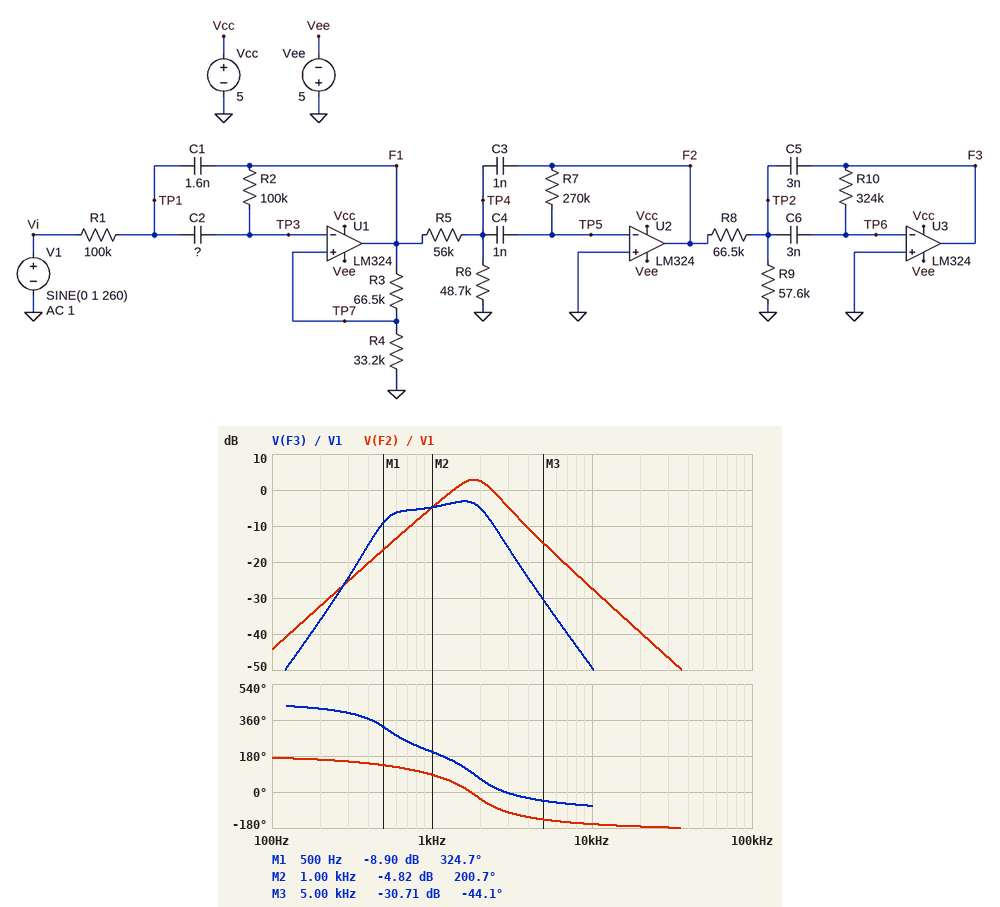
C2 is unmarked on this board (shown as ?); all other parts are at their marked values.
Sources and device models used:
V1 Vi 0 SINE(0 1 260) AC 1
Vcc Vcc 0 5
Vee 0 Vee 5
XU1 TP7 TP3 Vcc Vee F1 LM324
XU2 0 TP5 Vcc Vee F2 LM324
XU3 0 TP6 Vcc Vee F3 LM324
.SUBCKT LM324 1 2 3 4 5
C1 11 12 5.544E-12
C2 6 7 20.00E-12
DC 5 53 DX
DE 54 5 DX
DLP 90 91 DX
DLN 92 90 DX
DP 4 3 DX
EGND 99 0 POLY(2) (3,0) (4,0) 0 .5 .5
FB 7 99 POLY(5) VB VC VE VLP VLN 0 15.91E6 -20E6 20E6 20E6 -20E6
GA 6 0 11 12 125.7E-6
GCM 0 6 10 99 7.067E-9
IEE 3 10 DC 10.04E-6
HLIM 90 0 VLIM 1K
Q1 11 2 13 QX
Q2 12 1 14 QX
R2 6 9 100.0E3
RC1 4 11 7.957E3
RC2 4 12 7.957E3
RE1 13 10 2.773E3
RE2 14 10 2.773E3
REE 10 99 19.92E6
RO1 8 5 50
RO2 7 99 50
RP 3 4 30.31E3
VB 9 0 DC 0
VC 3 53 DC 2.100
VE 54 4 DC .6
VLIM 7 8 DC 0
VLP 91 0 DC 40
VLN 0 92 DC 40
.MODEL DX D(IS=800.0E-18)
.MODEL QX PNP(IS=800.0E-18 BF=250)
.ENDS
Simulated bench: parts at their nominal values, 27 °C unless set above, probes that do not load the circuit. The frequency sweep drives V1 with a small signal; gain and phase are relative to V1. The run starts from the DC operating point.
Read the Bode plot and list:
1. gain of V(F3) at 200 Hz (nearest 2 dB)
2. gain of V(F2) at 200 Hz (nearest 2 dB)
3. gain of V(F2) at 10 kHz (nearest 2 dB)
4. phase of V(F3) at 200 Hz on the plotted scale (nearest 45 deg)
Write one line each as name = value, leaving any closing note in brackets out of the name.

gain of V(F3) at 200 Hz = -36 dB
gain of V(F2) at 200 Hz = -32 dB
gain of V(F2) at 10 kHz = -28 dB
phase of V(F3) at 200 Hz on the plotted scale = 405 deg
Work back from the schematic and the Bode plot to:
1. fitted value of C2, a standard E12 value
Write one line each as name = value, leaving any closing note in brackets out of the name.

fitted value of C2, a standard E12 value = 820 pF
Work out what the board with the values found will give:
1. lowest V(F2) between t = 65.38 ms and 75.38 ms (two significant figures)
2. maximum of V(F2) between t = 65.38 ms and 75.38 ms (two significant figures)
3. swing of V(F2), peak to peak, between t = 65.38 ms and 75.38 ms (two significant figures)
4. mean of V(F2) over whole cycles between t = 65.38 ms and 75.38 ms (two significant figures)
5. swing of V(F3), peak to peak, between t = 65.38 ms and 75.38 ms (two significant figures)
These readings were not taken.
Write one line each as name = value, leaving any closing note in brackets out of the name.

lowest V(F2) between t = 65.38 ms and 75.38 ms = -46 mV
maximum of V(F2) between t = 65.38 ms and 75.38 ms = 36 mV
swing of V(F2), peak to peak, between t = 65.38 ms and 75.38 ms = 82 mV
mean of V(F2) over whole cycles between t = 65.38 ms and 75.38 ms = -5.4 mV
swing of V(F3), peak to peak, between t = 65.38 ms and 75.38 ms = 74 mV
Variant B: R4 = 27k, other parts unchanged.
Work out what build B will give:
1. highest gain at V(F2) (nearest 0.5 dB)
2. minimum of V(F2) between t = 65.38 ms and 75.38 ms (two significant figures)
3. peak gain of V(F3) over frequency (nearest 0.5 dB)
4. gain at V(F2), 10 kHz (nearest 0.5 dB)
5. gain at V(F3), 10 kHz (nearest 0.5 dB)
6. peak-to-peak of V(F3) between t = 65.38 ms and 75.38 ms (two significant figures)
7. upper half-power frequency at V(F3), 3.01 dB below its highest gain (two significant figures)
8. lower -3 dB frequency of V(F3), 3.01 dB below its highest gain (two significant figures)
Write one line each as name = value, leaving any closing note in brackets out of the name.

highest gain at V(F2) = 2.0 dB
minimum of V(F2) between t = 65.38 ms and 75.38 ms = -44 mV
peak gain of V(F3) over frequency = -4.0 dB
gain at V(F2), 10 kHz = -28.0 dB
gain at V(F3), 10 kHz = -50.0 dB
peak-to-peak of V(F3) between t = 65.38 ms and 75.38 ms = 69 mV
upper half-power frequency at V(F3), 3.01 dB below its highest gain = 2.1 kHz
lower -3 dB frequency of V(F3), 3.01 dB below its highest gain = 600 Hz
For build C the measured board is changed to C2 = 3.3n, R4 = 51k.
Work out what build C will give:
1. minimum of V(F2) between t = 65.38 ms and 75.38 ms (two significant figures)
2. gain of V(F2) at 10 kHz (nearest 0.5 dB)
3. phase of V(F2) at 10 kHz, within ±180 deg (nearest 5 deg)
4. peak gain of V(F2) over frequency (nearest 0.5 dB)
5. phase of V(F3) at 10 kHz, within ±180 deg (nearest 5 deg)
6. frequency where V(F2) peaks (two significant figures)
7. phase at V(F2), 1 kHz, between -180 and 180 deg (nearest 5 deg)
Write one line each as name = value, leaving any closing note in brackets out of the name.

minimum of V(F2) between t = 65.38 ms and 75.38 ms = -220 mV
gain of V(F2) at 10 kHz = -26.0 dB
phase of V(F2) at 10 kHz, within ±180 deg = -170 deg
peak gain of V(F2) over frequency = 8.0 dB
phase of V(F3) at 10 kHz, within ±180 deg = -80 deg
frequency where V(F2) peaks = 1.7 kHz
phase at V(F2), 1 kHz, between -180 and 180 deg = 30 deg
